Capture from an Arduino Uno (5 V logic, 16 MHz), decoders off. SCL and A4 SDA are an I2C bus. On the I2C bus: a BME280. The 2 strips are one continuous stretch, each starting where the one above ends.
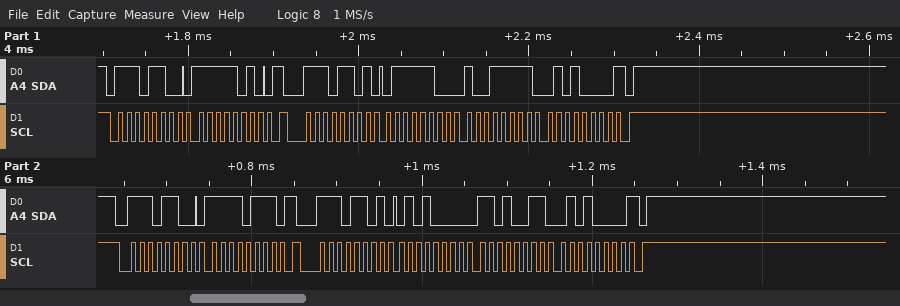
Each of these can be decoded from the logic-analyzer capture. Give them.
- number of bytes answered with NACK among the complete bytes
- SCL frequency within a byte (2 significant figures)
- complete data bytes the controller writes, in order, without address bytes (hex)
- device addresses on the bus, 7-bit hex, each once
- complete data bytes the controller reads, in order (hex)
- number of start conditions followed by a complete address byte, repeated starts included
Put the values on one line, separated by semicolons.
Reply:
2; 100 kHz; FA F7; 0x76; 7C 9F 50 50 D3 50; 4
